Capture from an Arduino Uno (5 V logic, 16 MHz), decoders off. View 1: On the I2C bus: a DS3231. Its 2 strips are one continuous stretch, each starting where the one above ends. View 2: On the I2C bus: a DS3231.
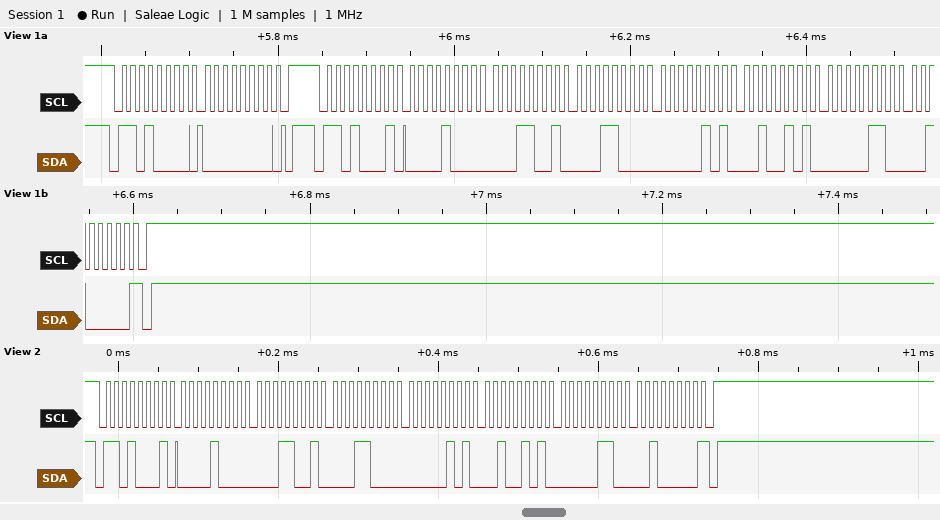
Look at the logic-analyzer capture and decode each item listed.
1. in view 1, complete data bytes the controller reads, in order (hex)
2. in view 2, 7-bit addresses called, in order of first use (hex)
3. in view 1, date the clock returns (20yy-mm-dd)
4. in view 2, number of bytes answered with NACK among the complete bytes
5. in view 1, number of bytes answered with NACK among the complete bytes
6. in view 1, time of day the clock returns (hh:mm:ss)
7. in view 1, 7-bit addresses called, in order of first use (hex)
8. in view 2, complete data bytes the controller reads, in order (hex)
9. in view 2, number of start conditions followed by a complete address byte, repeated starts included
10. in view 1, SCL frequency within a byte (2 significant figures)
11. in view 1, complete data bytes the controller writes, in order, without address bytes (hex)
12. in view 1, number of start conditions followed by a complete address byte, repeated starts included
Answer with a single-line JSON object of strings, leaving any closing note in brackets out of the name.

{"in view 1, complete data bytes the controller reads, in order": "08 19 18 05 25 06 20", "in view 2, 7-bit addresses called, in order of first use": "0x68", "in view 1, date the clock returns": "2020-06-25", "in view 2, number of bytes answered with NACK among the complete bytes": "1", "in view 1, number of bytes answered with NACK among the complete bytes": "1", "in view 1, time of day the clock returns": "18:19:08", "in view 1, 7-bit addresses called, in order of first use": "0x68", "in view 2, complete data bytes the controller reads, in order": "08 19 18 05 25 06 20", "in view 2, number of start conditions followed by a complete address byte, repeated starts included": "1", "in view 1, SCL frequency within a byte": "100 kHz", "in view 1, complete data bytes the controller writes, in order, without address bytes": "00", "in view 1, number of start conditions followed by a complete address byte, repeated starts included": "2"}
